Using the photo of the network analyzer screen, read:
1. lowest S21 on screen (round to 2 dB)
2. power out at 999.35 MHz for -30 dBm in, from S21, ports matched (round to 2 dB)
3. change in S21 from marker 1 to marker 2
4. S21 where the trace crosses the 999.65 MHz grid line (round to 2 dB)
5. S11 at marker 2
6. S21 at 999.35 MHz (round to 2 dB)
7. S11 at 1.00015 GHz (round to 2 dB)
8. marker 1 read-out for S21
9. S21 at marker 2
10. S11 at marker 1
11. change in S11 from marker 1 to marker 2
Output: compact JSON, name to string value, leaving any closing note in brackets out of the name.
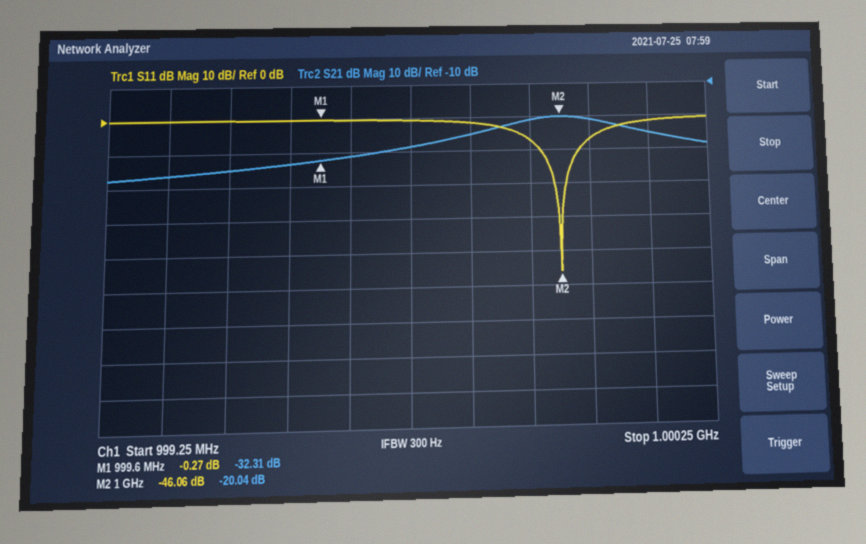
{"lowest S21 on screen": "-38 dB", "power out at 999.35 MHz for -30 dBm in, from S21, ports matched": "-66 dBm", "change in S21 from marker 1 to marker 2": "12.27 dB", "S21 where the trace crosses the 999.65 MHz grid line": "-32 dB", "S11 at marker 2": "-46.06 dB", "S21 at 999.35 MHz": "-36 dB", "S11 at 1.00015 GHz": "-2 dB", "marker 1 read-out for S21": "-32.31 dB", "S21 at marker 2": "-20.04 dB", "S11 at marker 1": "-0.27 dB", "change in S11 from marker 1 to marker 2": "-45.79 dB"}
